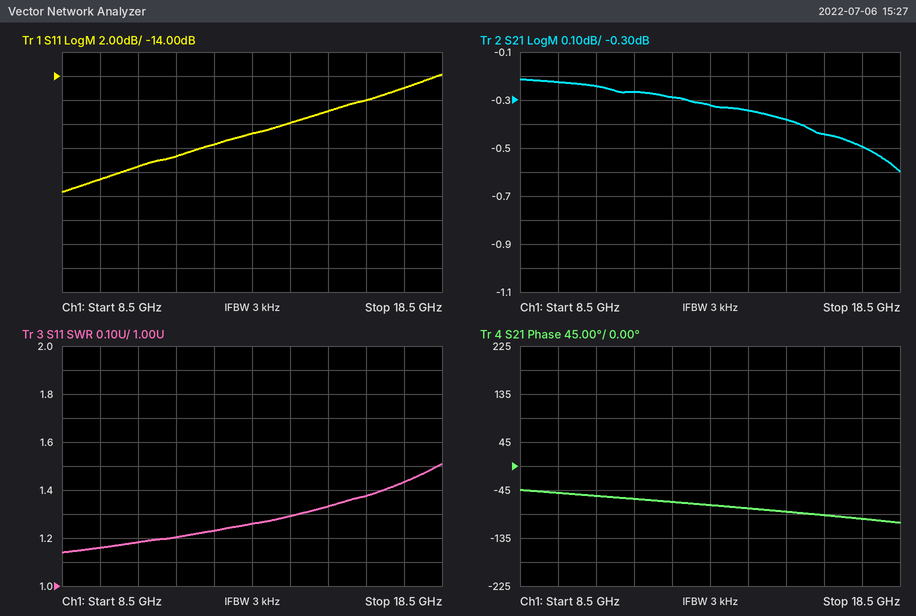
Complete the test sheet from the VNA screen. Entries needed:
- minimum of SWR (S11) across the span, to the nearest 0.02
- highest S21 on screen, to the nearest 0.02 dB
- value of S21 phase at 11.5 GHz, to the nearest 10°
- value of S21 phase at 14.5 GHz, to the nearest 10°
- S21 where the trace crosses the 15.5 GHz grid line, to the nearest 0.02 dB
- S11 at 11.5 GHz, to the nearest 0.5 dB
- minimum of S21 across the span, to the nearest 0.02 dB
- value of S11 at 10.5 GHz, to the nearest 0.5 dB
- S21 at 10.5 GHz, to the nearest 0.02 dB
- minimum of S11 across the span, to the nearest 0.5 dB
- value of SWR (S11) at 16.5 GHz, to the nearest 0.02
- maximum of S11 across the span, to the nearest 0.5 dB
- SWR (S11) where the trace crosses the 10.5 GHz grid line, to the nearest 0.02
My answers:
1.14
-0.22 dB
-60°
-80°
-0.38 dB
-20.5 dB
-0.60 dB
-21.5 dB
-0.24 dB
-23.5 dB
1.38
-14.0 dB
1.18
